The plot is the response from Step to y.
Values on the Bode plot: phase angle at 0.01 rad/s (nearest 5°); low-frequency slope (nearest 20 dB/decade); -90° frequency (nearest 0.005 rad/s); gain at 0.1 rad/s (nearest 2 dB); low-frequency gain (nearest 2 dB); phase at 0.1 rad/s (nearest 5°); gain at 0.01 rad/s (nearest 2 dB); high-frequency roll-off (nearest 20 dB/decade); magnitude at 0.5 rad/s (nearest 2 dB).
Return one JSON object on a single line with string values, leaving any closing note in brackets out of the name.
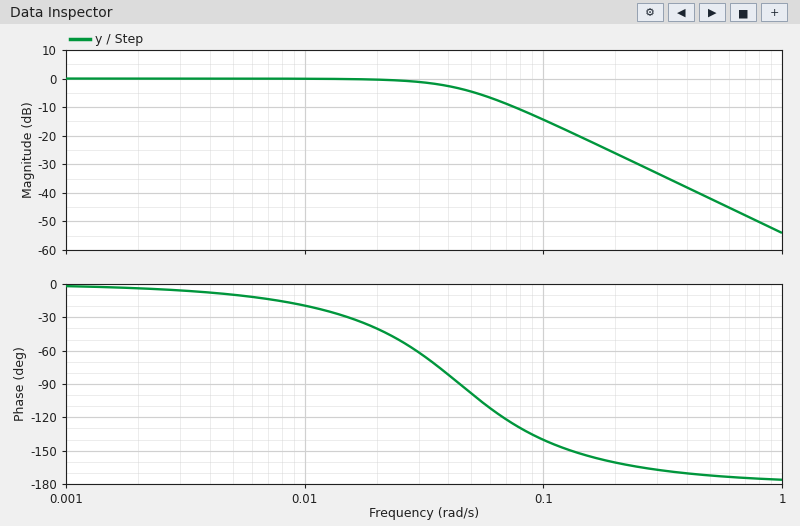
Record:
{"phase angle at 0.01 rad/s": "-20°", "low-frequency slope": "0 dB/decade", "-90° frequency": "0.045 rad/s", "gain at 0.1 rad/s": "-14 dB", "low-frequency gain": "0 dB", "phase at 0.1 rad/s": "-140°", "gain at 0.01 rad/s": "0 dB", "high-frequency roll-off": "-40 dB/decade", "magnitude at 0.5 rad/s": "-42 dB"}
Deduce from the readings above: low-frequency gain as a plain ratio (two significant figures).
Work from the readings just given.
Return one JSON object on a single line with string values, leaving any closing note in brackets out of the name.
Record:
{"low-frequency gain as a plain ratio": "1.0"}
